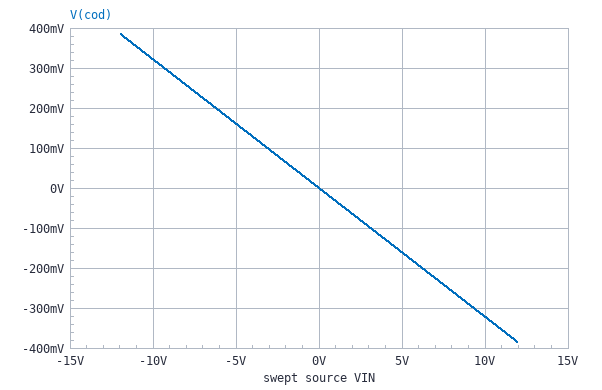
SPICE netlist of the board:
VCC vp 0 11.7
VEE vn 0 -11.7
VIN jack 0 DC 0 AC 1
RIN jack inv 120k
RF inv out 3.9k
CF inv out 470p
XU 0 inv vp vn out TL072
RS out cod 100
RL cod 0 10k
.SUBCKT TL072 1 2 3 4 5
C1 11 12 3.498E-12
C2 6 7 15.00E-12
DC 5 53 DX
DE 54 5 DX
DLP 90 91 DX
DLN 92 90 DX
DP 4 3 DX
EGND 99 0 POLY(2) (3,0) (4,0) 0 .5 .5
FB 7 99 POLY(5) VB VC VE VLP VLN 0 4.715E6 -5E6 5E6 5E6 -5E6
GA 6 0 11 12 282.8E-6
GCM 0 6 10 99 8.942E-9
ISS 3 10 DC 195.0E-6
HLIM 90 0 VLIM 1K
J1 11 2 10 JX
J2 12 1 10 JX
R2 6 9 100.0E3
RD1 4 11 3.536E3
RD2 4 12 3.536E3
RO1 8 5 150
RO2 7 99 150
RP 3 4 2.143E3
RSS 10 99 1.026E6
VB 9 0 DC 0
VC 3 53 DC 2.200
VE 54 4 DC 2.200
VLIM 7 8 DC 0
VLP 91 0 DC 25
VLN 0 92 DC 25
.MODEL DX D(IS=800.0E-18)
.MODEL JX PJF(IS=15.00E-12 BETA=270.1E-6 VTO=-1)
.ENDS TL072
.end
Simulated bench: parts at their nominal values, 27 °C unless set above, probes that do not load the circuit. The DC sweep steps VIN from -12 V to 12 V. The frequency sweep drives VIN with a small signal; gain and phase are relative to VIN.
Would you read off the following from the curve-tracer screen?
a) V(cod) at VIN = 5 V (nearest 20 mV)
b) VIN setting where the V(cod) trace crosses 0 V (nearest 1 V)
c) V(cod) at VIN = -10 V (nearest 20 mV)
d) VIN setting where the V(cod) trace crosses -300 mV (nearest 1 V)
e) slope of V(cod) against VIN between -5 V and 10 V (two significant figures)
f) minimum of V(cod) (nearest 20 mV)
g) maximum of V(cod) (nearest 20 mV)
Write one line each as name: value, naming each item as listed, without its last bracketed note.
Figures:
V(cod) at VIN = 5 V: -160 mV
VIN setting where the V(cod) trace crosses 0 V: 0 V
V(cod) at VIN = -10 V: 320 mV
VIN setting where the V(cod) trace crosses -300 mV: 9 V
slope of V(cod) against VIN between -5 V and 10 V: -0.032 V/V
minimum of V(cod): -380 mV
maximum of V(cod): 380 mV
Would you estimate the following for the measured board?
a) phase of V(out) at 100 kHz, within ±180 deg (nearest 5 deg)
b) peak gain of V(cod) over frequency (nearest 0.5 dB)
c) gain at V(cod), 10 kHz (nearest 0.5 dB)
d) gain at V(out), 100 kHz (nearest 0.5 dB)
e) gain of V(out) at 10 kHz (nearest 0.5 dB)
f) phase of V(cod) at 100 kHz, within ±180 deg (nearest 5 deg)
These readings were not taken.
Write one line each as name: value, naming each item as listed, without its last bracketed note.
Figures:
phase of V(out) at 100 kHz, within ±180 deg: 130 deg
peak gain of V(cod) over frequency: -30.0 dB
gain at V(cod), 10 kHz: -30.0 dB
gain at V(out), 100 kHz: -33.5 dB
gain of V(out) at 10 kHz: -30.0 dB
phase of V(cod) at 100 kHz, within ±180 deg: 130 deg
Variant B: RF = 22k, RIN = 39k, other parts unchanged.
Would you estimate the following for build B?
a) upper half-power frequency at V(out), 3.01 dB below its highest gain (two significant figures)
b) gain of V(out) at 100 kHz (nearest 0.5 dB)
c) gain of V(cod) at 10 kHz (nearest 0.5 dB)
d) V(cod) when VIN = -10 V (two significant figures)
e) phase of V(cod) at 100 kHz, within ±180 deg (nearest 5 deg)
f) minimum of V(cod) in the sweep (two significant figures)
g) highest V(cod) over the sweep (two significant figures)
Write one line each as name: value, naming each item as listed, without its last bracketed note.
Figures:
upper half-power frequency at V(out), 3.01 dB below its highest gain: 15 kHz
gain of V(out) at 100 kHz: -21.5 dB
gain of V(cod) at 10 kHz: -6.5 dB
V(cod) when VIN = -10 V: 5.6 V
phase of V(cod) at 100 kHz, within ±180 deg: 95 deg
minimum of V(cod) in the sweep: -6.7 V
highest V(cod) over the sweep: 6.7 V
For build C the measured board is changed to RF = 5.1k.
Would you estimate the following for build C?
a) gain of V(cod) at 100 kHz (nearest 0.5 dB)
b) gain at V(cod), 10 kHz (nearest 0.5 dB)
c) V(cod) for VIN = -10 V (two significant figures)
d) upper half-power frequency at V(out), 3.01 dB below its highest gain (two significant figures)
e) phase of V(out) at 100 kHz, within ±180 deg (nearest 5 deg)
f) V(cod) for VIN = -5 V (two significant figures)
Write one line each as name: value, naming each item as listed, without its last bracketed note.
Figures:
gain of V(cod) at 100 kHz: -32.5 dB
gain at V(cod), 10 kHz: -27.5 dB
V(cod) for VIN = -10 V: 420 mV
upper half-power frequency at V(out), 3.01 dB below its highest gain: 66 kHz
phase of V(out) at 100 kHz, within ±180 deg: 120 deg
V(cod) for VIN = -5 V: 210 mV
